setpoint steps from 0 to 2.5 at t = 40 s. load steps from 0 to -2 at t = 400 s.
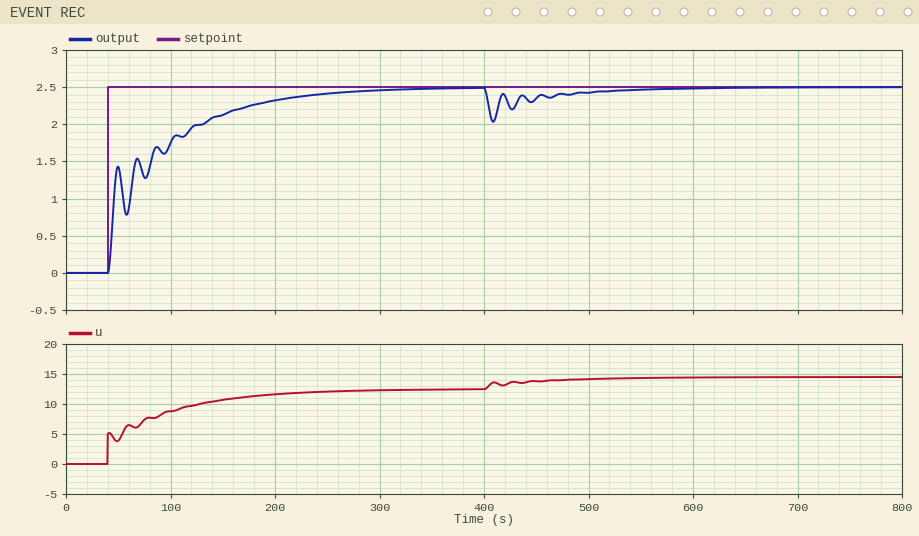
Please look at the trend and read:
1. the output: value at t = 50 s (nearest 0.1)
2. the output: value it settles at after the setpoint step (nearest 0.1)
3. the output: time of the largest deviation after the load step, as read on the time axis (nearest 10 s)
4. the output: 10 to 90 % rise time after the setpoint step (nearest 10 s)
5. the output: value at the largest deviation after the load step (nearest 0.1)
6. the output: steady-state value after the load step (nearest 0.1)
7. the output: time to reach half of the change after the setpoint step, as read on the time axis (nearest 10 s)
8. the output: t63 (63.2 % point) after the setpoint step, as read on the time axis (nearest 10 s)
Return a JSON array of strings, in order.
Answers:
["1.4", "2.5", "410 s", "130 s", "2.0", "2.5", "50 s", "80 s"]
